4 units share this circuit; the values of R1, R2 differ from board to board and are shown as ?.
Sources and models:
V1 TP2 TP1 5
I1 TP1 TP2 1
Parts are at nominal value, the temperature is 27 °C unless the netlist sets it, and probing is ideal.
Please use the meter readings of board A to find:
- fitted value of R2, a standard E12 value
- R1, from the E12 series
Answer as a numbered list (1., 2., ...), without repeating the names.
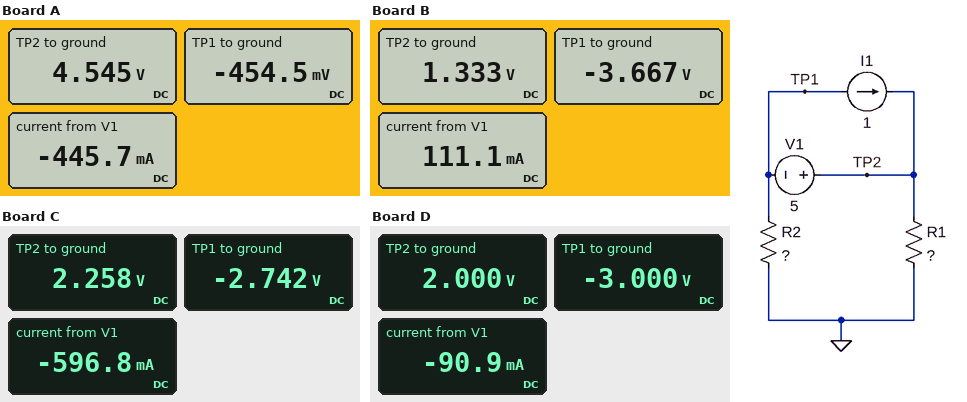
1. 0.82 Ω
2. 8.2 Ω
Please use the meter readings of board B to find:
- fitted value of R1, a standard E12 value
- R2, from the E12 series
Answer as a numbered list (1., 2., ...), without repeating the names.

1. 1.2 Ω
2. 3.3 Ω
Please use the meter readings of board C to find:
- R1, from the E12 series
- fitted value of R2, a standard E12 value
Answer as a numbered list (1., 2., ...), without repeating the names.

1. 5.6 Ω
2. 6.8 Ω
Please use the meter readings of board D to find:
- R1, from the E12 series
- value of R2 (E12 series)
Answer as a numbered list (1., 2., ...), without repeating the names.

1. 2.2 Ω
2. 3.3 Ω
